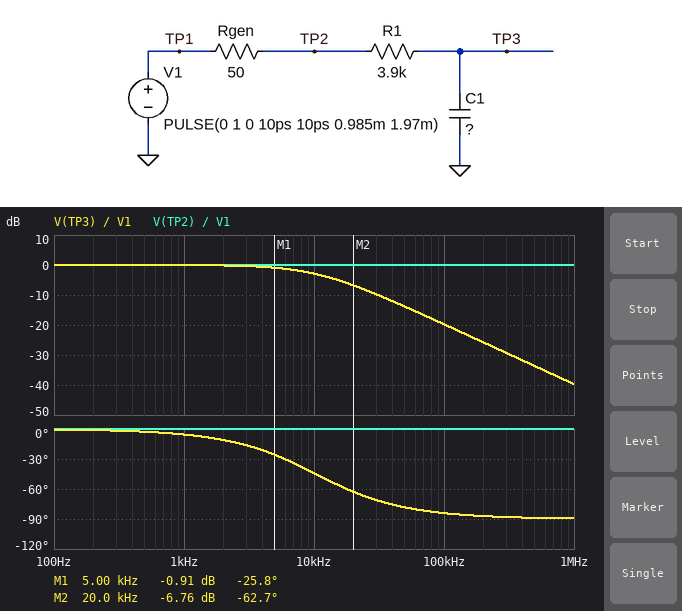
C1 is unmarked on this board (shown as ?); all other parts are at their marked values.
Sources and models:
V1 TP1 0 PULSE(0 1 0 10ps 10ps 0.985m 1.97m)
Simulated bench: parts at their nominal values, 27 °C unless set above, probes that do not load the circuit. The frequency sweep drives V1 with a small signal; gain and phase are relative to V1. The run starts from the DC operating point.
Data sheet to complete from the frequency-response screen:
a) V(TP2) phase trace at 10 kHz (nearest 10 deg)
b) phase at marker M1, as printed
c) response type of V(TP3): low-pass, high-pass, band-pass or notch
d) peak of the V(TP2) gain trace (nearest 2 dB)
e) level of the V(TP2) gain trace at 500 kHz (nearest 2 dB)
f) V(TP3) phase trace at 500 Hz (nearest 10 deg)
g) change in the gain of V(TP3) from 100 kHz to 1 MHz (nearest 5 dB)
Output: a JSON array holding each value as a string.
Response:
["0 deg", "-25.8 deg", "low-pass", "0 dB", "0 dB", "0 deg", "-20 dB"]
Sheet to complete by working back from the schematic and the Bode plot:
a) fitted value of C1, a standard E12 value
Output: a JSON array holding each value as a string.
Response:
["3.9 nF"]
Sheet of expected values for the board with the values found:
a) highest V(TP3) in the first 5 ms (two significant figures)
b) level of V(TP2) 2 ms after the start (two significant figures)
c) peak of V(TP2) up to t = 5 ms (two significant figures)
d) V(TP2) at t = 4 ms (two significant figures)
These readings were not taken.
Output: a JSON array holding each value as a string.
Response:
["1.0 V", "1.0 V", "1.0 V", "1.0 V"]
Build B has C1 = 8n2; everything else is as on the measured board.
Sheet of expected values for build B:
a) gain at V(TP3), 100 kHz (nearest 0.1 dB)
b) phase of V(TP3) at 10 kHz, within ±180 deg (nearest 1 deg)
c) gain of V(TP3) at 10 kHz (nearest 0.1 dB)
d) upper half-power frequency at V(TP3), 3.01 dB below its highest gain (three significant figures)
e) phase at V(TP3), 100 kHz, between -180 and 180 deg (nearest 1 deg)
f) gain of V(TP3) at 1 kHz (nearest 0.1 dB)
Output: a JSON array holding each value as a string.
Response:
["-26.2 dB", "-64 deg", "-7.1 dB", "4.91 kHz", "-87 deg", "-0.2 dB"]
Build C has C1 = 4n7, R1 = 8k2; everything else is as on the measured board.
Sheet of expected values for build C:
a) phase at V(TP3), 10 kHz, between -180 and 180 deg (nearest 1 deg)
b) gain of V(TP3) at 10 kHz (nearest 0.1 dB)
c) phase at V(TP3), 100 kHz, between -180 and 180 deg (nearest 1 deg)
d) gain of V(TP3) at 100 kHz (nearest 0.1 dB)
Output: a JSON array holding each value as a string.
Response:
["-68 deg", "-8.4 dB", "-88 deg", "-27.7 dB"]
